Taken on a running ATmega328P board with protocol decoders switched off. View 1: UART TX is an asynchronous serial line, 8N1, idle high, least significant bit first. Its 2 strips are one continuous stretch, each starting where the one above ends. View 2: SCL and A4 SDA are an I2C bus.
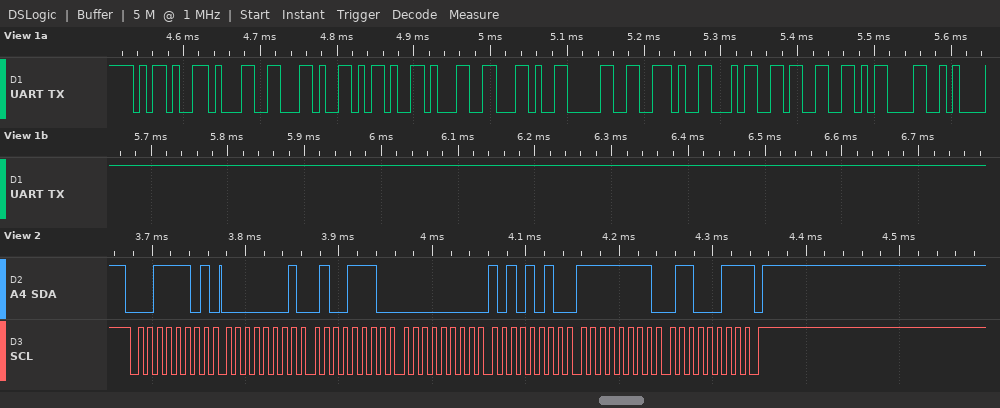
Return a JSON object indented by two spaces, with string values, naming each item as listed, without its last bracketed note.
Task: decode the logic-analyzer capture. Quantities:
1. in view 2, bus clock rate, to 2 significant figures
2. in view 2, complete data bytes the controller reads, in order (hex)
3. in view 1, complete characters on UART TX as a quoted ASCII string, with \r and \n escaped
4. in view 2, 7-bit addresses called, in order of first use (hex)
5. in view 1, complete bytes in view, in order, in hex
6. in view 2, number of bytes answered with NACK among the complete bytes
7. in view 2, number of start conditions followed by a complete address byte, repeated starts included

{
  "in view 2, bus clock rate, to 2 significant figures": "100 kHz",
  "in view 2, complete data bytes the controller reads, in order": "01 4E 00 AA FF 63",
  "in view 1, complete characters on UART TX as a quoted ASCII string, with \\r and \\n escaped": "\"-1,-1,0.43\\r\\n\"",
  "in view 2, 7-bit addresses called, in order of first use": "0x1E",
  "in view 1, complete bytes in view, in order, in hex": "2D 31 2C 2D 31 2C 30 2E 34 33 0D 0A",
  "in view 2, number of bytes answered with NACK among the complete bytes": "1",
  "in view 2, number of start conditions followed by a complete address byte, repeated starts included": "1"
}
